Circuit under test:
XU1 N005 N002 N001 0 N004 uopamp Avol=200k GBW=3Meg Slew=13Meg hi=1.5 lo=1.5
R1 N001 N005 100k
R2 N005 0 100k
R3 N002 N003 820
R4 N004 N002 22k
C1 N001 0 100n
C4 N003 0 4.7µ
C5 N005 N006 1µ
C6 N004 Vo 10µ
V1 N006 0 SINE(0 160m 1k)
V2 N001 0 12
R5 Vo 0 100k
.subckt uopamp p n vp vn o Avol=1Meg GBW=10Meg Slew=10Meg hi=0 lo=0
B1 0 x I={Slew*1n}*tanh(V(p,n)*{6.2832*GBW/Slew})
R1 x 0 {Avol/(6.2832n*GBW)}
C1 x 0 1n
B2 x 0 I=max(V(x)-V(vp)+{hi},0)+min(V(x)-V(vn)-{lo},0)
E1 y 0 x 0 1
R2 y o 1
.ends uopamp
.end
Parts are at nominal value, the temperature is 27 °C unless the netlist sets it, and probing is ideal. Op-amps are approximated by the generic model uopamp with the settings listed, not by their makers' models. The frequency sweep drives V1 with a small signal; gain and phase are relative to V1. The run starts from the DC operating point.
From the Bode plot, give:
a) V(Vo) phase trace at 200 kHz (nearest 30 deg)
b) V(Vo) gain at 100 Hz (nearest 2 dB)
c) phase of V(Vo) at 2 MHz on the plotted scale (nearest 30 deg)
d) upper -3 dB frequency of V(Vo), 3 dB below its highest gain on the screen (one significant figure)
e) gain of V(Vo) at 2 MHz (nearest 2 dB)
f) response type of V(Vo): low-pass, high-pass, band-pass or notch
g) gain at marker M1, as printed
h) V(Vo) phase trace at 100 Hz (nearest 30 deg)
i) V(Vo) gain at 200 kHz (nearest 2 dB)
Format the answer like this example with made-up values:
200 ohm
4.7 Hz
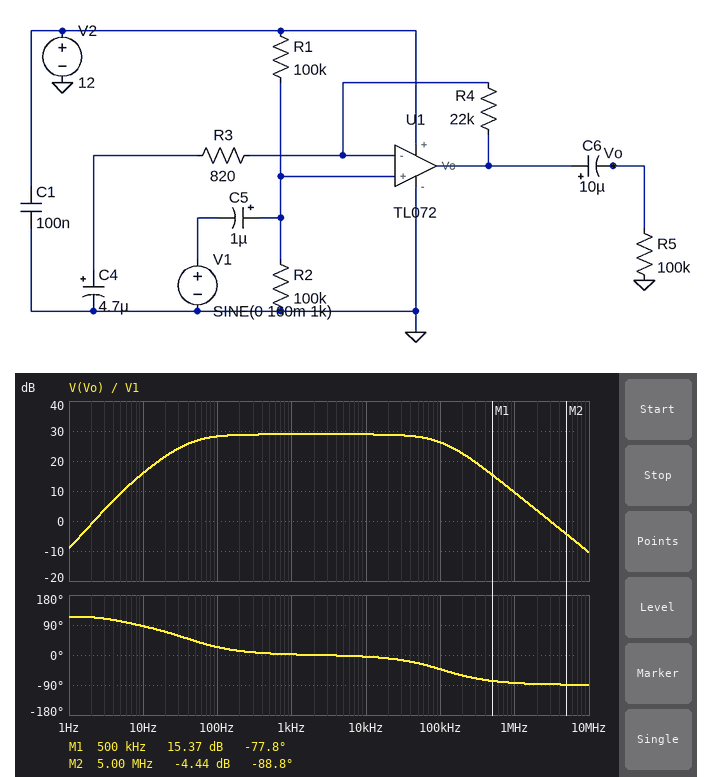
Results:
-60 deg
28 dB
-90 deg
100 kHz
4 dB
band-pass
15.37 dB
30 deg
22 dB
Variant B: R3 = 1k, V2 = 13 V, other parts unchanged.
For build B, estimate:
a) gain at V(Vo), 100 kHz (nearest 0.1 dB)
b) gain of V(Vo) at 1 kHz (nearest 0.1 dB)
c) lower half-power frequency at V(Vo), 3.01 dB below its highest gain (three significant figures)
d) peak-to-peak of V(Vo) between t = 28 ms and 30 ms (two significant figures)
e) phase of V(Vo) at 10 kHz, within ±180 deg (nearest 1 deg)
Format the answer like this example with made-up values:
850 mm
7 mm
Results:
25.2 dB
27.2 dB
34.1 Hz
7.4 V
-4 deg
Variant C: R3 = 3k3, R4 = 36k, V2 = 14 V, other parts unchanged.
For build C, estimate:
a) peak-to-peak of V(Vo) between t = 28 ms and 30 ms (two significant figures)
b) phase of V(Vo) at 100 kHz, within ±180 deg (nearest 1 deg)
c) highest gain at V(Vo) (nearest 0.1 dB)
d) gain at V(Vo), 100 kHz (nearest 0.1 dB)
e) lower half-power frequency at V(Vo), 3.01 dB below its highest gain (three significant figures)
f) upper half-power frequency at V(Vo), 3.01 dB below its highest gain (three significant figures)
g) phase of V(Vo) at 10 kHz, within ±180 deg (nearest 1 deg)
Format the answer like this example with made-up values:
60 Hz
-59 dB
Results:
3.8 V
-22 deg
21.5 dB
20.9 dB
11.1 Hz
252 kHz
-2 deg
